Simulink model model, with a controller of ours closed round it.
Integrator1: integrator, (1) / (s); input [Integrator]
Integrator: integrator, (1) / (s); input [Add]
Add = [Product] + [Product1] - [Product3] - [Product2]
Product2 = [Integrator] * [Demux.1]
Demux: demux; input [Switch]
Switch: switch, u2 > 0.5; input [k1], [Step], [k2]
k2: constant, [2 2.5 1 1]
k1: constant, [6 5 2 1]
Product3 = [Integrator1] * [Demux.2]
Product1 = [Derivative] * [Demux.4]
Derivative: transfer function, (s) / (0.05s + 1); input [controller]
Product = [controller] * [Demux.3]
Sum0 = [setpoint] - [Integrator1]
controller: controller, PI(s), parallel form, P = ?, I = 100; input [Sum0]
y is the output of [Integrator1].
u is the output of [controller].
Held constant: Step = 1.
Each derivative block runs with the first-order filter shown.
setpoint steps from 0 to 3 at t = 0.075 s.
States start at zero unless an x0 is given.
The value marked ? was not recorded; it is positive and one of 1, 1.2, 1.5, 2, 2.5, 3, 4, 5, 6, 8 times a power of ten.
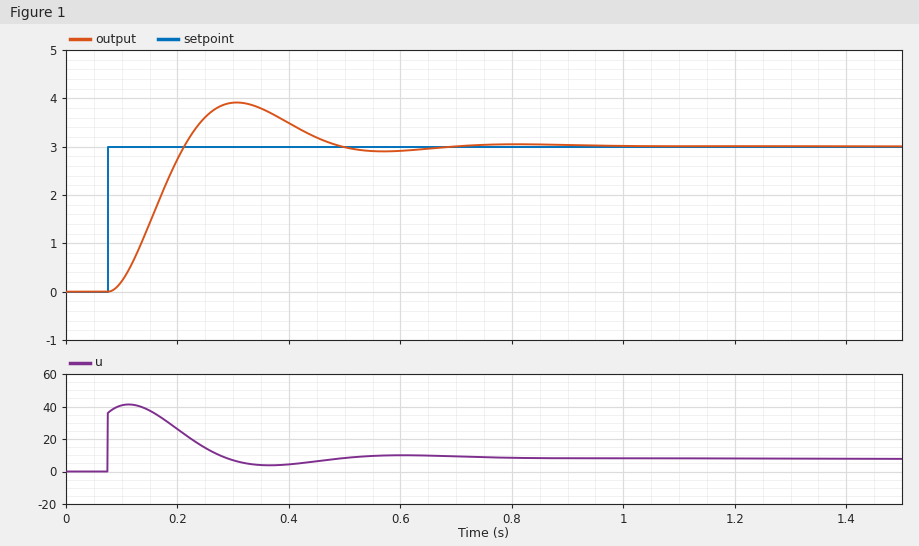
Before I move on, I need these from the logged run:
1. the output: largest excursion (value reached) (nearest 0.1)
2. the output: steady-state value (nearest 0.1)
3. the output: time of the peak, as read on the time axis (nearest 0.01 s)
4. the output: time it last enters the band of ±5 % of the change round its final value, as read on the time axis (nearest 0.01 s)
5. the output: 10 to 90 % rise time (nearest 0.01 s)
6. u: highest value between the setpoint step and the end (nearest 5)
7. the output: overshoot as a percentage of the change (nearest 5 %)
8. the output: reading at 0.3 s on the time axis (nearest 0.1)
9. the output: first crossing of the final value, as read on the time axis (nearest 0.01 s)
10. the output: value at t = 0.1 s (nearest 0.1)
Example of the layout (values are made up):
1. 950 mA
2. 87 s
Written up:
1. 3.9
2. 3.0
3. 0.31 s
4. 0.46 s
5. 0.09 s
6. 40
7. 30 %
8. 3.9
9. 0.21 s
10. 0.2
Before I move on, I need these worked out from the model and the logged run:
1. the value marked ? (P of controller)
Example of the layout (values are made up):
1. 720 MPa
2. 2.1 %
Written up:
1. 12
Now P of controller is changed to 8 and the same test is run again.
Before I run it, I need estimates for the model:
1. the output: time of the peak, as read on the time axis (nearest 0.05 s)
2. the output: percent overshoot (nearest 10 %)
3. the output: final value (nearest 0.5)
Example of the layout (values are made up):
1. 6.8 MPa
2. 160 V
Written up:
1. 0.35 s
2. 40 %
3. 3.0
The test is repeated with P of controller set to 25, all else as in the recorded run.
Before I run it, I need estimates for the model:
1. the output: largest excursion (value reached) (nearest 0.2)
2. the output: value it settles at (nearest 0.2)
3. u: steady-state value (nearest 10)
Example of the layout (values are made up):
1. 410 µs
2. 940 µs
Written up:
1. 3.6
2. 3.0
3. 10
